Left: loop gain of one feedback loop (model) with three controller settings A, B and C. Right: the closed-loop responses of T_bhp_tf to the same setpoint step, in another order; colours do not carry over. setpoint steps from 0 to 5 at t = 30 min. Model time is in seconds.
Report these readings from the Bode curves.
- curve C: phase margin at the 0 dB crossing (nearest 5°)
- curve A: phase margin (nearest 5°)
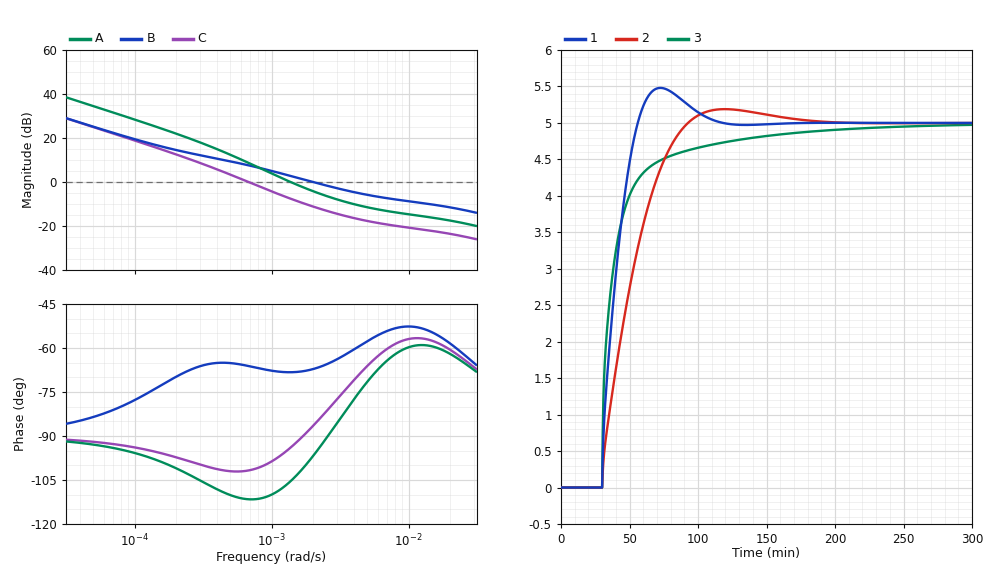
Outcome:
80°
75°
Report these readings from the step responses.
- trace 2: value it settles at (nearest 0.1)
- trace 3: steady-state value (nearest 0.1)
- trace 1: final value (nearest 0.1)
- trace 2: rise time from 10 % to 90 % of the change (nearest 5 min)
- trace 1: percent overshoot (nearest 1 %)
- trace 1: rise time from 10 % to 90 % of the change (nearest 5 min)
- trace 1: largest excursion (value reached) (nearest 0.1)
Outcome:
5.0
5.0
5.0
45 min
10 %
20 min
5.5
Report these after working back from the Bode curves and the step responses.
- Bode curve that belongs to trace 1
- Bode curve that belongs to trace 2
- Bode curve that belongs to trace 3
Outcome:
A
C
B
